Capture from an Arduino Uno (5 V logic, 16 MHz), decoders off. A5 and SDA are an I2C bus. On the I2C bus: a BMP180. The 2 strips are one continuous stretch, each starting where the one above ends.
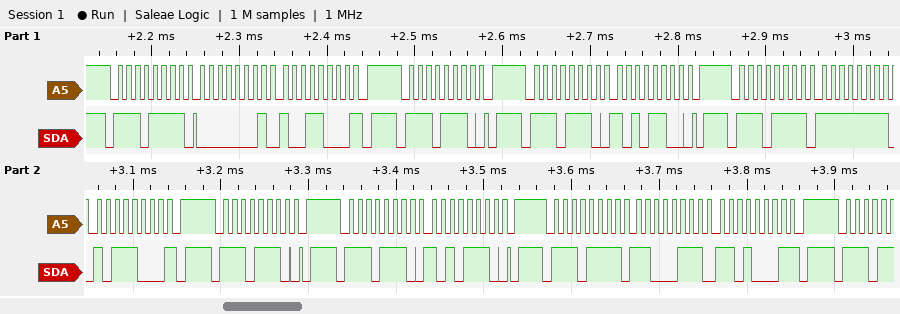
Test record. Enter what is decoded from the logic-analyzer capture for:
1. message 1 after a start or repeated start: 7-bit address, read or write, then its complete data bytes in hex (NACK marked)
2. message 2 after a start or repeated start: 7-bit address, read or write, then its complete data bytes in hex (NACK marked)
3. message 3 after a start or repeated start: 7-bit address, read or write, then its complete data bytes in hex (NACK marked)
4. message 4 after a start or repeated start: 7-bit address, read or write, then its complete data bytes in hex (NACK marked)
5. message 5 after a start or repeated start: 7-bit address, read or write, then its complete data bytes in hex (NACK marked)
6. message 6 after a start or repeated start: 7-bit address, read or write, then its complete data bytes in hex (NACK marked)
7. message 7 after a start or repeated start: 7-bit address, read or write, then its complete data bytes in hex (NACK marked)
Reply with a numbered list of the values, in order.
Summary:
1. 0x77 read: 01 98 NACK
2. 0x77 write
3. 0x77 write: AC
4. 0x77 read: FF B8 NACK
5. 0x77 write
6. 0x77 write: AE
7. 0x77 read: C7 D1 NACK
